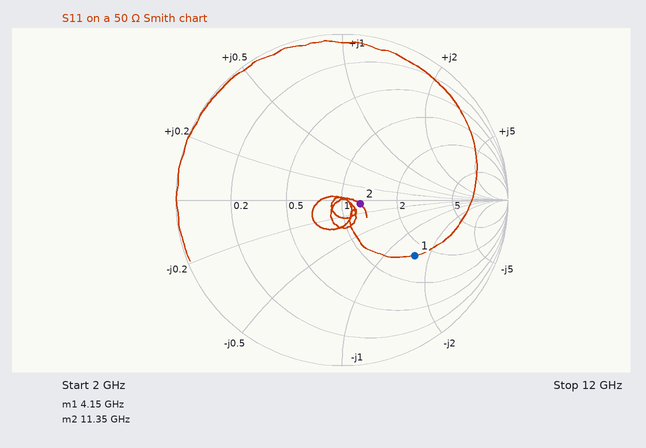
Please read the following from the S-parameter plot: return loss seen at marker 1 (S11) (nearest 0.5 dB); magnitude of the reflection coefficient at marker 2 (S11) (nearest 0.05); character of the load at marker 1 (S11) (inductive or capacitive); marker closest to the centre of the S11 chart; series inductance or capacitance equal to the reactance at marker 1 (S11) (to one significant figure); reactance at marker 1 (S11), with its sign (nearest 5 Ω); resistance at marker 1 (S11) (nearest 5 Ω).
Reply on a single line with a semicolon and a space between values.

5.0 dB; 0.10; capacitive; marker 2; 500 fF; -80 Ω; 80 Ω
